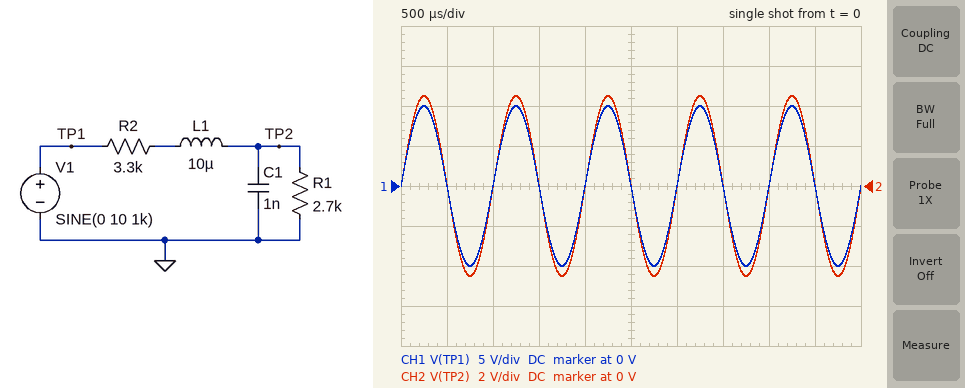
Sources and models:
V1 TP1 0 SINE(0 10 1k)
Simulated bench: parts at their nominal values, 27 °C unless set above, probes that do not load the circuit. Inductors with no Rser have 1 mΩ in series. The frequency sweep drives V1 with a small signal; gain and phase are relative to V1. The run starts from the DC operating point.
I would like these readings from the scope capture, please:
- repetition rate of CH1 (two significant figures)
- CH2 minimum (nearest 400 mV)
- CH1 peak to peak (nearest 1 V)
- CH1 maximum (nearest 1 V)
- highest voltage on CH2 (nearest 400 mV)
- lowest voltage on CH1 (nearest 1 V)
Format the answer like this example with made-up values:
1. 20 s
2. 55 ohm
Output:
1. 1.0 kHz
2. -4.4 V
3. 20 V
4. 10 V
5. 4.4 V
6. -10 V
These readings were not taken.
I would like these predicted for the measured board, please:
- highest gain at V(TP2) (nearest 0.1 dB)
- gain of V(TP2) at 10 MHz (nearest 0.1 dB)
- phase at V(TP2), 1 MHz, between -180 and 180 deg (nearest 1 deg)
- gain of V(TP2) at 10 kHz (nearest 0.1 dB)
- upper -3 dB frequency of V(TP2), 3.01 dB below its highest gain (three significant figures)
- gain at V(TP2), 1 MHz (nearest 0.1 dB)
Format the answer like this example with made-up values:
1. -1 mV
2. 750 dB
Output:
1. -6.9 dB
2. -46.5 dB
3. -85 deg
4. -7.0 dB
5. 107 kHz
6. -26.4 dB
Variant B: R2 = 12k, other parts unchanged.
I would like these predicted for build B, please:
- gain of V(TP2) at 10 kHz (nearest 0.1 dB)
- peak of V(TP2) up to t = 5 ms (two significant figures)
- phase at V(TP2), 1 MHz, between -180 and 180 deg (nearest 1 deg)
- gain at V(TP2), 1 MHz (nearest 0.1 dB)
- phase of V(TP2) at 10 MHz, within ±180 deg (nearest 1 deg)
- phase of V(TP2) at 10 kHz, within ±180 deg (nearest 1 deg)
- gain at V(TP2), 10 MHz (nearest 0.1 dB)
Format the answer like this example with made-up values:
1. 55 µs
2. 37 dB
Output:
1. -14.8 dB
2. 1.8 V
3. -86 deg
4. -37.6 dB
5. -93 deg
6. -8 deg
7. -57.6 dB
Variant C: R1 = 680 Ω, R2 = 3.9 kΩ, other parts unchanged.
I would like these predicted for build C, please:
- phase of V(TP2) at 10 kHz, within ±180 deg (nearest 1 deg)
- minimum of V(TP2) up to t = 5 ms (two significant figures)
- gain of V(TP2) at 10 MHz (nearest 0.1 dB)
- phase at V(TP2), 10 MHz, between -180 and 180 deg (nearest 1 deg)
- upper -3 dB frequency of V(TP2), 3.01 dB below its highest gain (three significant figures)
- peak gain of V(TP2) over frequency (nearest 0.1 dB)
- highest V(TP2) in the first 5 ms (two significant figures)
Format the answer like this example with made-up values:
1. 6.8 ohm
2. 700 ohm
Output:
1. -2 deg
2. -1.5 V
3. -47.9 dB
4. -98 deg
5. 275 kHz
6. -16.6 dB
7. 1.5 V
